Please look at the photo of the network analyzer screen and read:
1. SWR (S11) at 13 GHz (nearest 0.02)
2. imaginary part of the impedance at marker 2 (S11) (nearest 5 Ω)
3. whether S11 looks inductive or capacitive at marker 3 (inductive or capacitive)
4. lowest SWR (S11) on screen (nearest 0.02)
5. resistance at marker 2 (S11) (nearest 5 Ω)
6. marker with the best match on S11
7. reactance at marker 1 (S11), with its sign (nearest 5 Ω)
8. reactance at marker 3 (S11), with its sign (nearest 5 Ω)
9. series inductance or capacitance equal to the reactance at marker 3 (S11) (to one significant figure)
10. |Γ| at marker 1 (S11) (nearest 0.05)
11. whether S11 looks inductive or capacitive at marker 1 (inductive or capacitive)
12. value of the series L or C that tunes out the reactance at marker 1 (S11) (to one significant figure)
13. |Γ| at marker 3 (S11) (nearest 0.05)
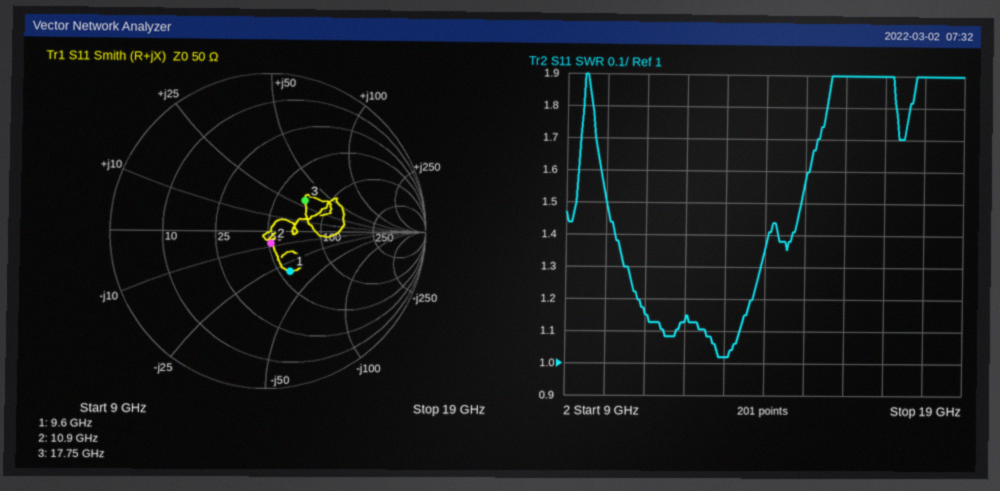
1.02
-10 Ω
inductive
1.02
50 Ω
marker 2
-30 Ω
+30 Ω
300 pH
0.30
capacitive
500 pH
0.30
